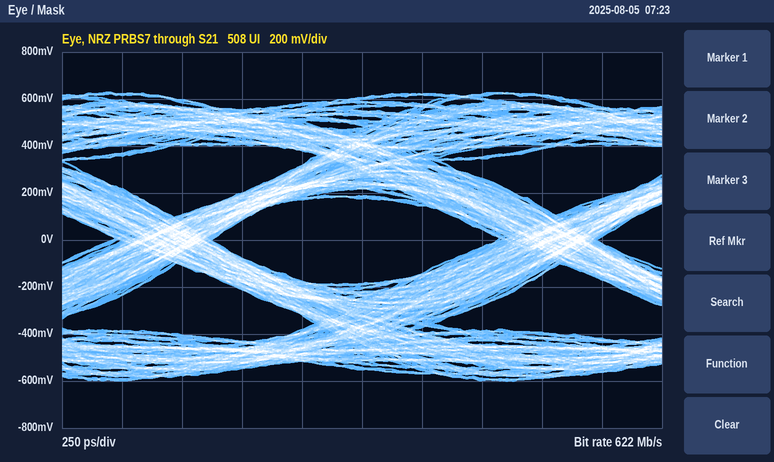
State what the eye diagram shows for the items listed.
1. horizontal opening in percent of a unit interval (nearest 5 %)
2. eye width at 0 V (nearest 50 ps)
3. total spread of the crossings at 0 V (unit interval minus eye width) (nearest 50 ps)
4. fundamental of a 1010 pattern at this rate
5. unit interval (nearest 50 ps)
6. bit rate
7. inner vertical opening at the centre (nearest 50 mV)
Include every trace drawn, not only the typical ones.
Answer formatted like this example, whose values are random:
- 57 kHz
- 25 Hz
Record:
- 75 %
- 1.20 ns
- 400 ps
- 311 MHz
- 1.60 ns
- 622 Mb/s
- 350 mV
